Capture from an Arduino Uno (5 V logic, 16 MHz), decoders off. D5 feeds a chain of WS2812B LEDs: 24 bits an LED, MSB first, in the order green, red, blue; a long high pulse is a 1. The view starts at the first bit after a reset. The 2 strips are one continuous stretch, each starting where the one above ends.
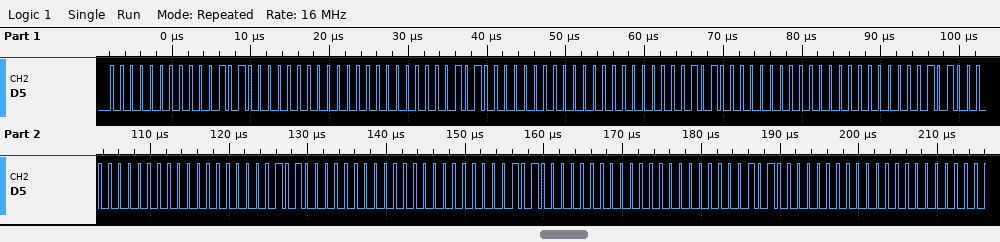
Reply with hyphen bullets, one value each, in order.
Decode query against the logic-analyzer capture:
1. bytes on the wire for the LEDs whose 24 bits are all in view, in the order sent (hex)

- 00 14 00 00 14 00 00 14 00 00 14 00 00 14 00 00 14 00 00 14 00
